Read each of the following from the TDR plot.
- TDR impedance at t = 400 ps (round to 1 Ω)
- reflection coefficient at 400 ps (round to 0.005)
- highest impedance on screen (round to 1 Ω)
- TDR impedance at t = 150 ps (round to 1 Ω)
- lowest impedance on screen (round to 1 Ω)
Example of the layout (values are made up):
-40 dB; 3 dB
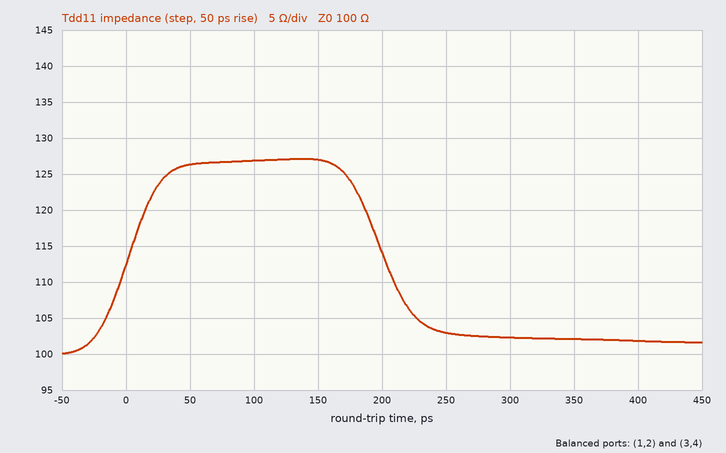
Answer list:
102 Ω; +0.010; 127 Ω; 127 Ω; 100 Ω
